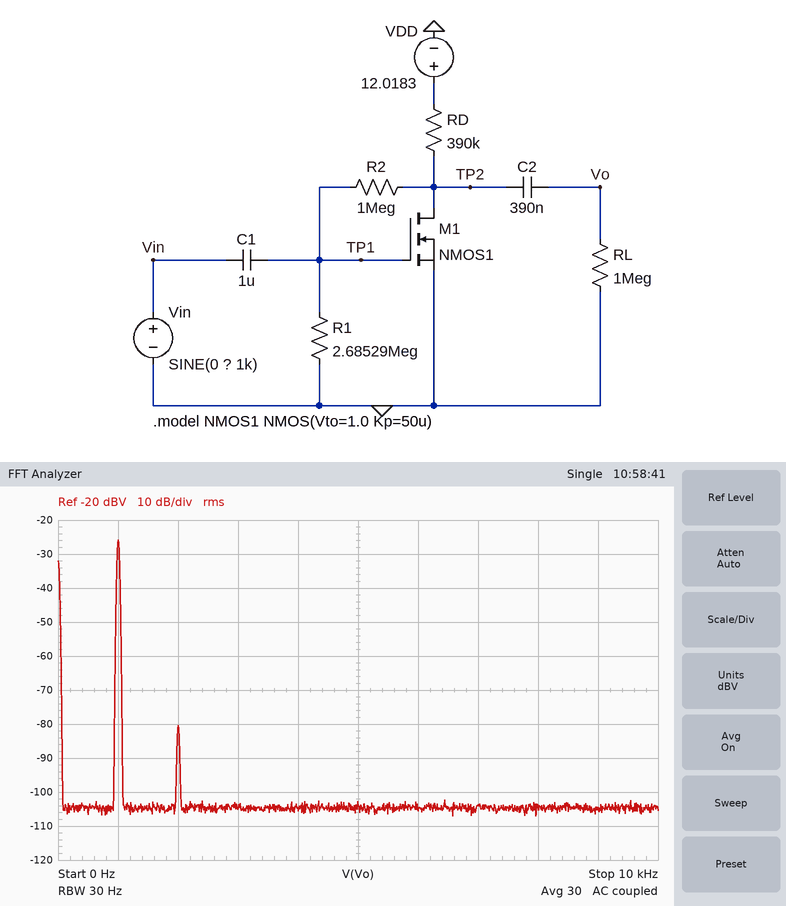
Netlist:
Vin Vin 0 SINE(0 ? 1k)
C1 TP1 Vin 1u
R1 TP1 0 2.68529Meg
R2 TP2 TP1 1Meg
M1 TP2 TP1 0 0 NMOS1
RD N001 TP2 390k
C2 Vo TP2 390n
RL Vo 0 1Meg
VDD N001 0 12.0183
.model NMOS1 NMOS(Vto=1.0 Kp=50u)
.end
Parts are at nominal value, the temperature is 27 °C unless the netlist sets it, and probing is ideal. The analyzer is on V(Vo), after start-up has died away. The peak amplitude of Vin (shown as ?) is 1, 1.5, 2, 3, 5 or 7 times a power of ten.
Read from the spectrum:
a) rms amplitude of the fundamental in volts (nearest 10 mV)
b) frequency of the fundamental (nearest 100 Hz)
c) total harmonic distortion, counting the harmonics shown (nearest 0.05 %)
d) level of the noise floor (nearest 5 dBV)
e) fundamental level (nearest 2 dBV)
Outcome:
50 mV
1.0 kHz
0.20 %
-105 dBV
-26 dBV
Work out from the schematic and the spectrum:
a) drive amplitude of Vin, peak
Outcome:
7 mV
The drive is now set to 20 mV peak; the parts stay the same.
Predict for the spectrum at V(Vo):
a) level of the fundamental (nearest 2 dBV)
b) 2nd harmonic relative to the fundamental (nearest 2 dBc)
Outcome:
-16 dBV
-46 dBc
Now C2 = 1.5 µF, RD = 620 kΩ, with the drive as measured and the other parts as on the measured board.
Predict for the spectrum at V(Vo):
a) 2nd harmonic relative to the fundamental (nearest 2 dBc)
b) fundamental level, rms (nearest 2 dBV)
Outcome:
-52 dBc
-26 dBV
